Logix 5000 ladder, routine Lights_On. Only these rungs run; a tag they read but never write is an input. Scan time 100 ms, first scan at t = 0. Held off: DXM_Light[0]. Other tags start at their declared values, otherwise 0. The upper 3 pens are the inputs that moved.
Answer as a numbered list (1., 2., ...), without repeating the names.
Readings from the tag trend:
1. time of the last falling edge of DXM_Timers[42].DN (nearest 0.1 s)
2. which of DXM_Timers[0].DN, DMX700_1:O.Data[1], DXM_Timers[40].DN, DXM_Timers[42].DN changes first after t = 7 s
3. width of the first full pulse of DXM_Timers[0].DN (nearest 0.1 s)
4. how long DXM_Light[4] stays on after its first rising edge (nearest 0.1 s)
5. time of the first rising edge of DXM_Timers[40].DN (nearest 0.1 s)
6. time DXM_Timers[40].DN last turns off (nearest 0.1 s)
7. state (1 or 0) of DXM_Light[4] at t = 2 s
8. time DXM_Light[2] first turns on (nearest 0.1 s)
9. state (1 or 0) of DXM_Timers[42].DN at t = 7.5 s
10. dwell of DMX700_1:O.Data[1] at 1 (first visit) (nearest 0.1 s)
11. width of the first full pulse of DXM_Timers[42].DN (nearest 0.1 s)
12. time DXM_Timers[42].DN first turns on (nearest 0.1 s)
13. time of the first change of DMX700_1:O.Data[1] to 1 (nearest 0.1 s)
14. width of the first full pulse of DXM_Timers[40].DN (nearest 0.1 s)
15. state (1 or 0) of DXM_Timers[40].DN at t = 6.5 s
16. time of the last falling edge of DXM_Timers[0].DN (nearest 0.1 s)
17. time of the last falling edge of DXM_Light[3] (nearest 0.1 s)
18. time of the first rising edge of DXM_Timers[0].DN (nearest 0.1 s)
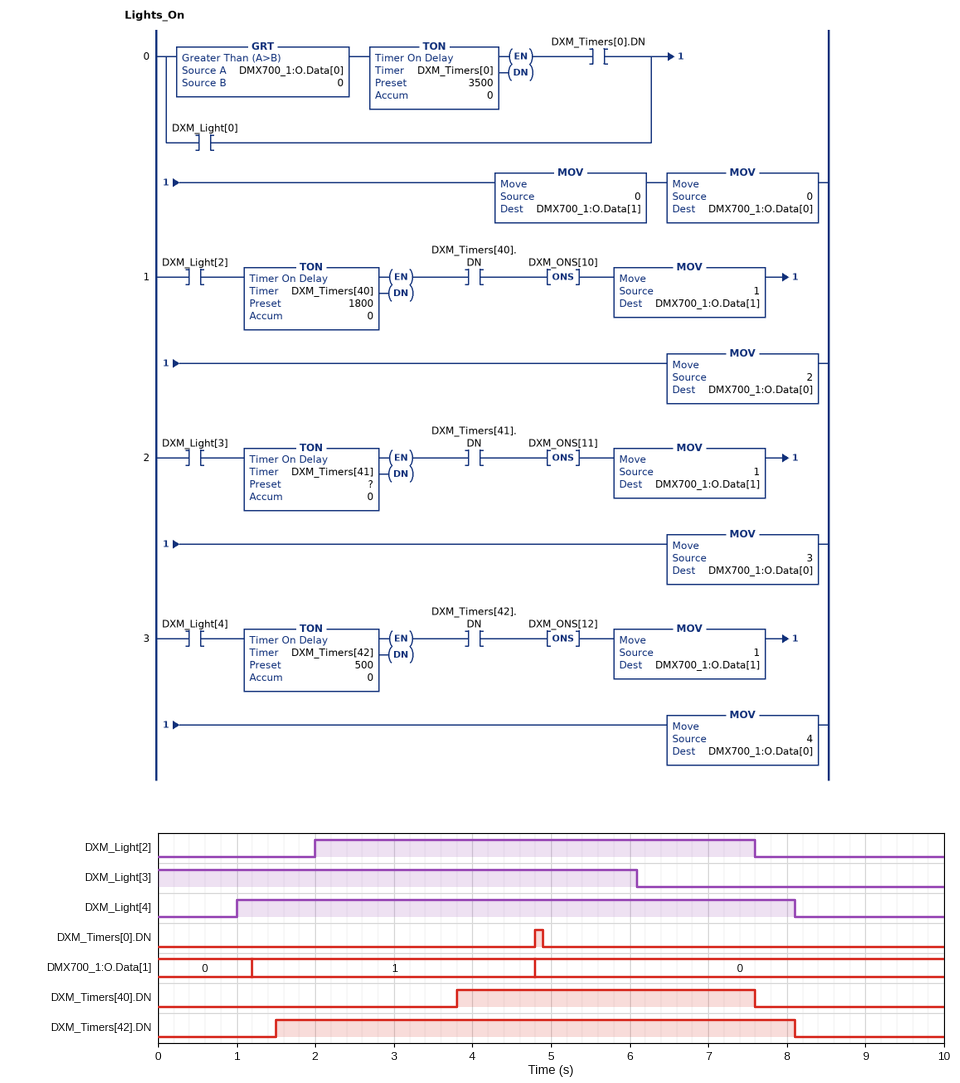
1. 8.1 s
2. DXM_Timers[40].DN
3. 0.1 s
4. 7.1 s
5. 3.8 s
6. 7.6 s
7. 1
8. 2.0 s
9. 1
10. 3.6 s
11. 6.6 s
12. 1.5 s
13. 1.2 s
14. 3.8 s
15. 1
16. 4.9 s
17. 6.1 s
18. 4.8 s
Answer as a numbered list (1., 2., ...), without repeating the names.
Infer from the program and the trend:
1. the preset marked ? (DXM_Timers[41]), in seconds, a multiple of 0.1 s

1. 1.2 s
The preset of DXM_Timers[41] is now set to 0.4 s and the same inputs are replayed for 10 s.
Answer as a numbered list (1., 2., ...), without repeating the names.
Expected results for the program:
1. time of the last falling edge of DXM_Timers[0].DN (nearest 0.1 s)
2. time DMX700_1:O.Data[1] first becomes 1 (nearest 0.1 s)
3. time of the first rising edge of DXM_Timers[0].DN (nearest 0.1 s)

1. 4.1 s
2. 0.4 s
3. 4.0 s
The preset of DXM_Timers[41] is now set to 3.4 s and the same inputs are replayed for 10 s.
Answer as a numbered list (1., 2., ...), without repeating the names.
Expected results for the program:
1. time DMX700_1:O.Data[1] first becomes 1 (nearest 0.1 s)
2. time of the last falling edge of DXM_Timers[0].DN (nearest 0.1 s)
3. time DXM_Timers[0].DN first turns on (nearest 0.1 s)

1. 1.5 s
2. 5.2 s
3. 5.1 s
